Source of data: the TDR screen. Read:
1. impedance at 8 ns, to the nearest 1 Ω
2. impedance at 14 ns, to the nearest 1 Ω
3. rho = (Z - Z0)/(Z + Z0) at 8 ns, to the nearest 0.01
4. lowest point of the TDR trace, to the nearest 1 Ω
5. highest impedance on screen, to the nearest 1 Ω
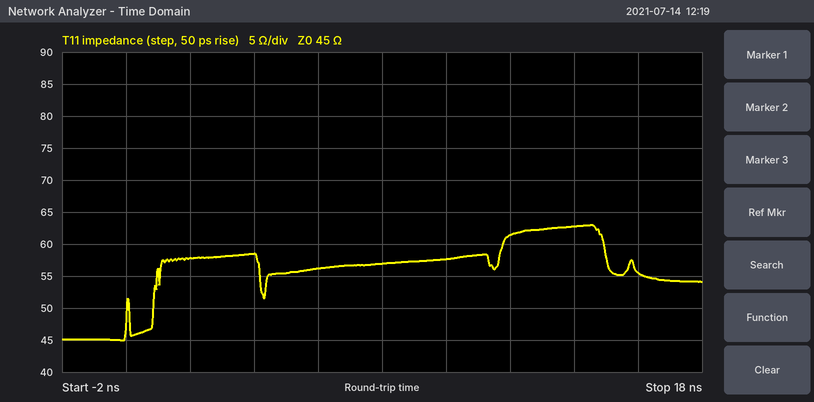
57 Ω
63 Ω
+0.12
45 Ω
63 Ω
